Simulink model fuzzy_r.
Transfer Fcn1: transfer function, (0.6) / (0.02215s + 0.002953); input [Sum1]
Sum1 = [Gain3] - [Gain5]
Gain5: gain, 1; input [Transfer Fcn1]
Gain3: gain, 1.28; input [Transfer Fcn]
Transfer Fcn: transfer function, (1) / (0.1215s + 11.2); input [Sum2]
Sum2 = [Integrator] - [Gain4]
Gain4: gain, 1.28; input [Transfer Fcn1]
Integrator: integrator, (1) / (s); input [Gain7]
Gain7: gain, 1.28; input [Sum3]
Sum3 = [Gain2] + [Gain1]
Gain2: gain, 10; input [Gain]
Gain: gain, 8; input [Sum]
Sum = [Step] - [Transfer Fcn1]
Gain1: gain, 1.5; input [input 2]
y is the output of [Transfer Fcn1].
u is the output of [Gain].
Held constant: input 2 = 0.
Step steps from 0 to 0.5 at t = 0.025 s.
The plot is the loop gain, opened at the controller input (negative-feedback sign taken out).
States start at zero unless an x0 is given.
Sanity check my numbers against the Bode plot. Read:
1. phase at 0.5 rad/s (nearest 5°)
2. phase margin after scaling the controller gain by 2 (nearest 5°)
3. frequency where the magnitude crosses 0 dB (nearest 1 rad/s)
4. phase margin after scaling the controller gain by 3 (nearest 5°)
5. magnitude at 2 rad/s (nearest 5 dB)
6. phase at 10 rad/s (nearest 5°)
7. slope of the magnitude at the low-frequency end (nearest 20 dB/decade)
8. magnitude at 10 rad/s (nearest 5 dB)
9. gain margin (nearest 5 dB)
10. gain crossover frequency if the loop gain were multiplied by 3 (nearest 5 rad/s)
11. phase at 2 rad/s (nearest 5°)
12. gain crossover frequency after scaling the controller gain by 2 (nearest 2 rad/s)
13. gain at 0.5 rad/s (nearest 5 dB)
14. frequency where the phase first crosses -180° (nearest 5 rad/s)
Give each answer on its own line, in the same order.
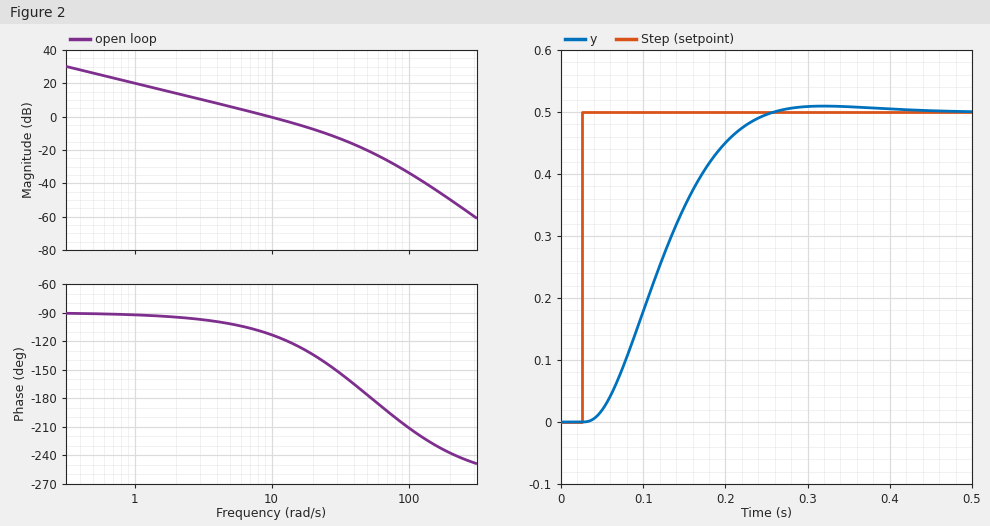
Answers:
-90°
50°
10 rad/s
40°
15 dB
-115°
-20 dB/decade
0 dB
20 dB
25 rad/s
-95°
18 rad/s
25 dB
55 rad/s
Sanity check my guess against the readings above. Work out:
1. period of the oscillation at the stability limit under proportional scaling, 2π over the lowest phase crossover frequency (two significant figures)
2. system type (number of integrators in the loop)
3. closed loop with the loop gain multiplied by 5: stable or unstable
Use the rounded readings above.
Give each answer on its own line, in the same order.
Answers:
0.11 s
1
stable
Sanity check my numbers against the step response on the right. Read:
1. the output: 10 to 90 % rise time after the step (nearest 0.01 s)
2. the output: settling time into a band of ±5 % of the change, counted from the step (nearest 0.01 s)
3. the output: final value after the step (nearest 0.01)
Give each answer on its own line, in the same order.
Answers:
0.14 s
0.20 s
0.50
